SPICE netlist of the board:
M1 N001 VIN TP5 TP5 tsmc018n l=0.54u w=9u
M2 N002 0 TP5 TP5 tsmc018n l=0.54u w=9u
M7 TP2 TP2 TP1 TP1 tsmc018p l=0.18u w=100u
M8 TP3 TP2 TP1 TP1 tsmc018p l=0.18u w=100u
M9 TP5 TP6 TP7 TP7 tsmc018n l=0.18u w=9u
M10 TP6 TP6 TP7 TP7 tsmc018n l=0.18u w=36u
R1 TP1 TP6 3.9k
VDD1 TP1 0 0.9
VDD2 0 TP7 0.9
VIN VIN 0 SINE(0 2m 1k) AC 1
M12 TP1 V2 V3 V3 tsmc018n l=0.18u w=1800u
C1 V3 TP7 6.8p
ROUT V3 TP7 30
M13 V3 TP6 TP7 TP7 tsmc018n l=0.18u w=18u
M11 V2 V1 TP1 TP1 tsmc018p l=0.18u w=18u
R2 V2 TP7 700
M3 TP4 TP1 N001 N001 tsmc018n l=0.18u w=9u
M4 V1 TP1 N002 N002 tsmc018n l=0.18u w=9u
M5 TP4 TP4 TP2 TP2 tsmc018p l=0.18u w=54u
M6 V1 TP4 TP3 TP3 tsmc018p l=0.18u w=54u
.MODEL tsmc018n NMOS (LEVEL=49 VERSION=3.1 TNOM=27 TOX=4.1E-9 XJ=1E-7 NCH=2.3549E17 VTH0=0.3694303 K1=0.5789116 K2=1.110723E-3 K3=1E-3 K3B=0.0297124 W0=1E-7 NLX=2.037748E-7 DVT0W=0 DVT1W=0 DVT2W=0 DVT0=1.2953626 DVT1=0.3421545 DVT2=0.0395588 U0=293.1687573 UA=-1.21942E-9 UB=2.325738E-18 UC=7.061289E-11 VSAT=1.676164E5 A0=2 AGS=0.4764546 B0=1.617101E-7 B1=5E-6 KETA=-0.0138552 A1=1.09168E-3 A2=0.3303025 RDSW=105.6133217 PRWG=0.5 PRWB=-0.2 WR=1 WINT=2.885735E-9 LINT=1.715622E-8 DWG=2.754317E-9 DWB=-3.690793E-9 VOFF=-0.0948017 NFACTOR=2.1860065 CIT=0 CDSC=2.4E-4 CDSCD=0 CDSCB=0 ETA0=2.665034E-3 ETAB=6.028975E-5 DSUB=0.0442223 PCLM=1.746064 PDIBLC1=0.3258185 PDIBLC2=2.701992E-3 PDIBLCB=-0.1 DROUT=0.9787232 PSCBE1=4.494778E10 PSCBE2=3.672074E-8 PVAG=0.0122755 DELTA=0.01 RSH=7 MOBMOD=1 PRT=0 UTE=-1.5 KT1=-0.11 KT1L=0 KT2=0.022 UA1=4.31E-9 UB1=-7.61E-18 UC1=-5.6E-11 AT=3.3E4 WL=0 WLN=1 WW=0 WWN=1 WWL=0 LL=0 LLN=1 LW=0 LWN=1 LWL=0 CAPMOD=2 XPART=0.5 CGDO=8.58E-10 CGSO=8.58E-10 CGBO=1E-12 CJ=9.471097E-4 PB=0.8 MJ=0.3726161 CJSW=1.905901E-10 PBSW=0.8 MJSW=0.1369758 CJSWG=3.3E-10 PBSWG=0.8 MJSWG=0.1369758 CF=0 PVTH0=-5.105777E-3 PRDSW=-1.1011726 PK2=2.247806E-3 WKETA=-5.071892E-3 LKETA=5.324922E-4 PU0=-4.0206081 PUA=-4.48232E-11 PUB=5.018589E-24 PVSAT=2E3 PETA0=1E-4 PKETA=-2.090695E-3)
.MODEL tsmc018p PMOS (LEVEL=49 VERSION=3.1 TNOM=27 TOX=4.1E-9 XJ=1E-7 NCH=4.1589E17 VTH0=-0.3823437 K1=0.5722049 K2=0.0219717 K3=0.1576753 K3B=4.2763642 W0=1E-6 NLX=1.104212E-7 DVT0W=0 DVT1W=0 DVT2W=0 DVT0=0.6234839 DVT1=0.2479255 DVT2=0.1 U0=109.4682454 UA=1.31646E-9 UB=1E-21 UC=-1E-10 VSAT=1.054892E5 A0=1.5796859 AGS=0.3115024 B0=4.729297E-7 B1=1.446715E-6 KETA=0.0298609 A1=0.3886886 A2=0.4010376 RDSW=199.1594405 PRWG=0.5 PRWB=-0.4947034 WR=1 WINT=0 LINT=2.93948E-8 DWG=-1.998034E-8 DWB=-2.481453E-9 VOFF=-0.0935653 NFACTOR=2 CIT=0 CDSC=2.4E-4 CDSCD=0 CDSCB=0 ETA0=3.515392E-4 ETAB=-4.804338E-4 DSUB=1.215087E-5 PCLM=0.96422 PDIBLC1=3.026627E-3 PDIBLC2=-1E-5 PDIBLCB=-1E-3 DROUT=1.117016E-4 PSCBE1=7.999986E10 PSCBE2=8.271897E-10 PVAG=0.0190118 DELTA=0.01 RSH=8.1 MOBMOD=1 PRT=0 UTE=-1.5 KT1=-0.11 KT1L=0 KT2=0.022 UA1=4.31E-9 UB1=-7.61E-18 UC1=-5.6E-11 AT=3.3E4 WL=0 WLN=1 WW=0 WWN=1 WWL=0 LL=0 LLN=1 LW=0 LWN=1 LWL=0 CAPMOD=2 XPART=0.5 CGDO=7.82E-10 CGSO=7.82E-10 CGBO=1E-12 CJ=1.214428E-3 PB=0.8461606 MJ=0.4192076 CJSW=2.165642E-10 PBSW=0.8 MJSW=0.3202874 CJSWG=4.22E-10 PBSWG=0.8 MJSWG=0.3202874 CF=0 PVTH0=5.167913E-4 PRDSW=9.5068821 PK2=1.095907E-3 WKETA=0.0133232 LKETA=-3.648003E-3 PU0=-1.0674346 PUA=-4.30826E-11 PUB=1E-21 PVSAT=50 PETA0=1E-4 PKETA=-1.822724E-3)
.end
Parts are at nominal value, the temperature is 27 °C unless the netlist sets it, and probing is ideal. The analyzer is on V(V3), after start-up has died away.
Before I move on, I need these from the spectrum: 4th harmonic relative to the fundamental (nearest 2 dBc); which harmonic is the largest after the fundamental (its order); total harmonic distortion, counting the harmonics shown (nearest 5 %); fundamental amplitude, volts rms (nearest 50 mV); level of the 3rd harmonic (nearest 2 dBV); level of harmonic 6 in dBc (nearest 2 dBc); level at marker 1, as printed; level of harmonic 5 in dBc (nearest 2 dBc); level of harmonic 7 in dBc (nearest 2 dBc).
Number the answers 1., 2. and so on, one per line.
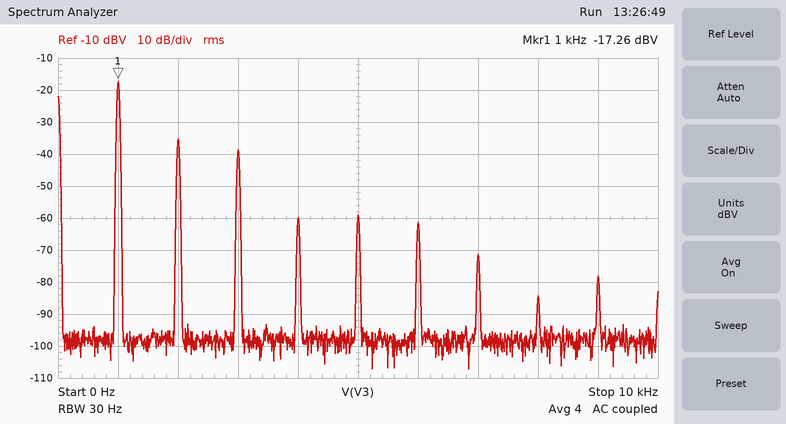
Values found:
1. -42 dBc
2. 2
3. 15 %
4. 150 mV
5. -38 dBV
6. -44 dBc
7. -17.26 dBV
8. -42 dBc
9. -54 dBc
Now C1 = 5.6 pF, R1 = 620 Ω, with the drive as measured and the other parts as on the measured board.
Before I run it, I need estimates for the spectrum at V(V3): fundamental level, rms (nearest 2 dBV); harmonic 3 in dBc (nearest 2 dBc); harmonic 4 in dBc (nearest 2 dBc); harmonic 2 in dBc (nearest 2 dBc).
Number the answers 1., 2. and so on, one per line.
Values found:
1. -20 dBV
2. -58 dBc
3. -56 dBc
4. -20 dBc
